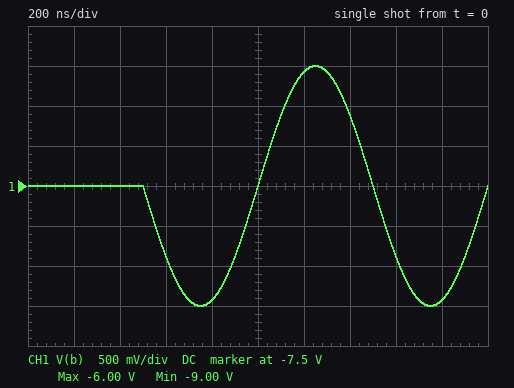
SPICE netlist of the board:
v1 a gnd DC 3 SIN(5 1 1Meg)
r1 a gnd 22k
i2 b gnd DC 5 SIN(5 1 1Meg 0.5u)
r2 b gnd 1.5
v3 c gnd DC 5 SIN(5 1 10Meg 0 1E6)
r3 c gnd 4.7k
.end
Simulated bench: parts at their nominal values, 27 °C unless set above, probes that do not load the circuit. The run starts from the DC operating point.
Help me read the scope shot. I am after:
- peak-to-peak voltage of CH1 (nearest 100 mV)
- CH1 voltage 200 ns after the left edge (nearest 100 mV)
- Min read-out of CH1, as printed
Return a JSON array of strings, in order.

["3.0 V", "-7.5 V", "-9.00 V"]
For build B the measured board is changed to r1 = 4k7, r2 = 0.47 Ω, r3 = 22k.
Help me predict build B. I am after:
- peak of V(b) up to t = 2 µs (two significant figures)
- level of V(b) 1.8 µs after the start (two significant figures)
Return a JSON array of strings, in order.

["-1.9 V", "-2.8 V"]
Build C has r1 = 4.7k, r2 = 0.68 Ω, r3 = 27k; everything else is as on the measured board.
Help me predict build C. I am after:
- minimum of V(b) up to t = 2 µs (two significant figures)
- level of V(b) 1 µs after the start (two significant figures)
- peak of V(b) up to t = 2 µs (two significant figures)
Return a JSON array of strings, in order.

["-4.1 V", "-3.4 V", "-2.7 V"]
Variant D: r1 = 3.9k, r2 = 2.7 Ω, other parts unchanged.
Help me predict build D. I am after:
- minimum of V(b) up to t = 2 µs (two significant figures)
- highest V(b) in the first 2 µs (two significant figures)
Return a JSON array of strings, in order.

["-16 V", "-11 V"]
